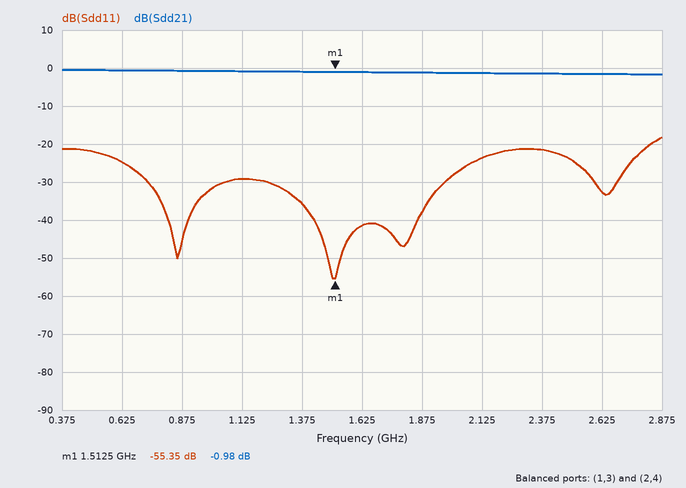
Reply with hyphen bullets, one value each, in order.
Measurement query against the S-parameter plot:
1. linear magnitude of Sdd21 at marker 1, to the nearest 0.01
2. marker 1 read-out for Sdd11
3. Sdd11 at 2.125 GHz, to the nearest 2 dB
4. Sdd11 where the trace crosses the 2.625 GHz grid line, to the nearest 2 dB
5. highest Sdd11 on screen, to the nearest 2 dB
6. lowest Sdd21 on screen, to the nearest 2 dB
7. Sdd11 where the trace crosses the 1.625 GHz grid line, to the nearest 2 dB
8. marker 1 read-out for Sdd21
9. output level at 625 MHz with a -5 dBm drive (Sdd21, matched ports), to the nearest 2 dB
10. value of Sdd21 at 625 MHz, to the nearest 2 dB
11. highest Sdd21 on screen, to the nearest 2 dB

- 0.89
- -55.35 dB
- -24 dB
- -32 dB
- -18 dB
- -2 dB
- -42 dB
- -0.98 dB
- -6 dBm
- 0 dB
- 0 dB
